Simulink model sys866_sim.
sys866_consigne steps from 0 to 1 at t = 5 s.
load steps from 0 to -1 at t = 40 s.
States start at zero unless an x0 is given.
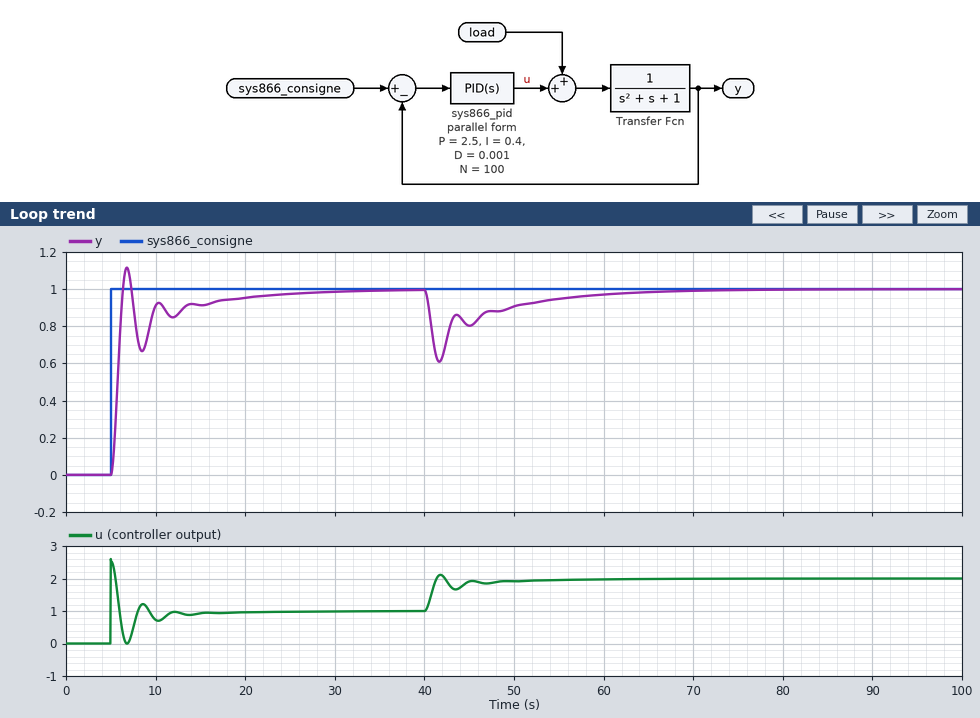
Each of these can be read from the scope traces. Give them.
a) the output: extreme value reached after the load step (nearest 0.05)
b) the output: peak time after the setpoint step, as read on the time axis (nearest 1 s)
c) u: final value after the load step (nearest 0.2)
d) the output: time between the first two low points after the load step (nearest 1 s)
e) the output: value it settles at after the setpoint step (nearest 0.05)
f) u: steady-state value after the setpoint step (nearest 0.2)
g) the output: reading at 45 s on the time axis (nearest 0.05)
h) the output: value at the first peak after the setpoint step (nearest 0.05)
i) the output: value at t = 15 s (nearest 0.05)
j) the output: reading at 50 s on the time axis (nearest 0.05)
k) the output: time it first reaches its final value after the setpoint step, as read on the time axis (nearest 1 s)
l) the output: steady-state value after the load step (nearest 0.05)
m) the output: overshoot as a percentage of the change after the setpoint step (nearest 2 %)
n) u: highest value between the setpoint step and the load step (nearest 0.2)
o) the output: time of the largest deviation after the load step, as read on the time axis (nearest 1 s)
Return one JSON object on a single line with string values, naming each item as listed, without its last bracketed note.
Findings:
{"the output: extreme value reached after the load step": "0.60", "the output: peak time after the setpoint step, as read on the time axis": "7 s", "u: final value after the load step": "2.0", "the output: time between the first two low points after the load step": "3 s", "the output: value it settles at after the setpoint step": "1.00", "u: steady-state value after the setpoint step": "1.0", "the output: reading at 45 s on the time axis": "0.80", "the output: value at the first peak after the setpoint step": "1.10", "the output: value at t = 15 s": "0.90", "the output: reading at 50 s on the time axis": "0.90", "the output: time it first reaches its final value after the setpoint step, as read on the time axis": "6 s", "the output: steady-state value after the load step": "1.00", "the output: overshoot as a percentage of the change after the setpoint step": "12 %", "u: highest value between the setpoint step and the load step": "2.6", "the output: time of the largest deviation after the load step, as read on the time axis": "42 s"}
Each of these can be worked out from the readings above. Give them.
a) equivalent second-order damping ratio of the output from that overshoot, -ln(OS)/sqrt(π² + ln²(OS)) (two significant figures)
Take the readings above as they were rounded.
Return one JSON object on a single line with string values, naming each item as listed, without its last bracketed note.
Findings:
{"equivalent second-order damping ratio of the output from that overshoot, -ln(OS)/sqrt(π² + ln²(OS))": "0.56"}
